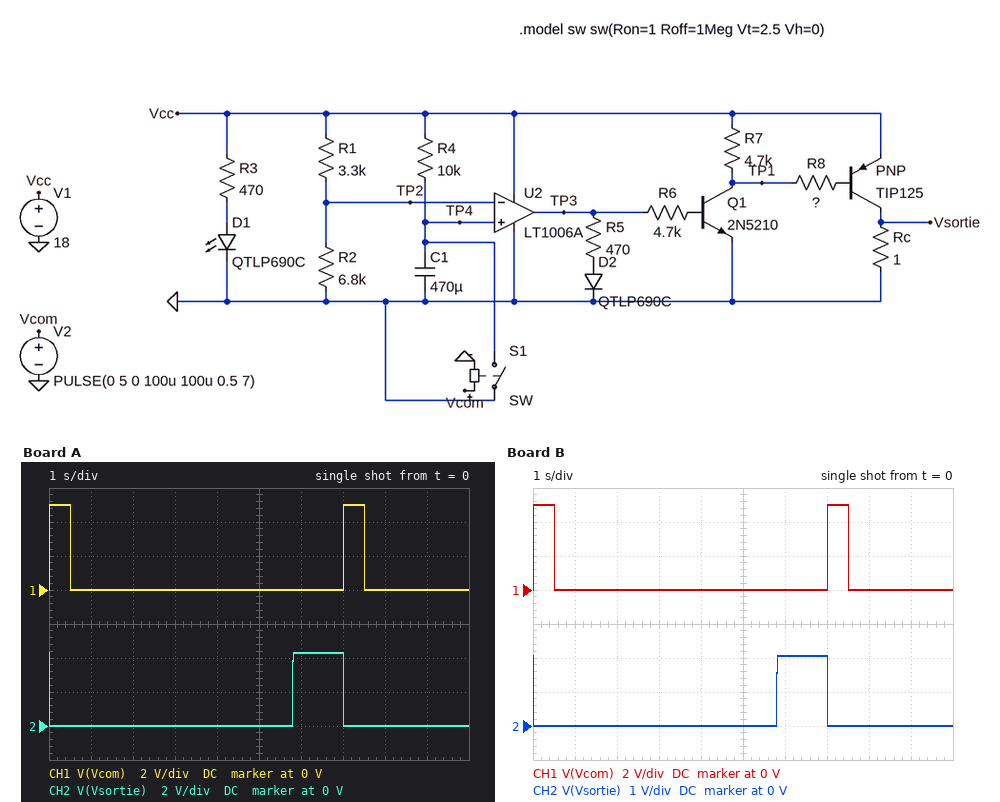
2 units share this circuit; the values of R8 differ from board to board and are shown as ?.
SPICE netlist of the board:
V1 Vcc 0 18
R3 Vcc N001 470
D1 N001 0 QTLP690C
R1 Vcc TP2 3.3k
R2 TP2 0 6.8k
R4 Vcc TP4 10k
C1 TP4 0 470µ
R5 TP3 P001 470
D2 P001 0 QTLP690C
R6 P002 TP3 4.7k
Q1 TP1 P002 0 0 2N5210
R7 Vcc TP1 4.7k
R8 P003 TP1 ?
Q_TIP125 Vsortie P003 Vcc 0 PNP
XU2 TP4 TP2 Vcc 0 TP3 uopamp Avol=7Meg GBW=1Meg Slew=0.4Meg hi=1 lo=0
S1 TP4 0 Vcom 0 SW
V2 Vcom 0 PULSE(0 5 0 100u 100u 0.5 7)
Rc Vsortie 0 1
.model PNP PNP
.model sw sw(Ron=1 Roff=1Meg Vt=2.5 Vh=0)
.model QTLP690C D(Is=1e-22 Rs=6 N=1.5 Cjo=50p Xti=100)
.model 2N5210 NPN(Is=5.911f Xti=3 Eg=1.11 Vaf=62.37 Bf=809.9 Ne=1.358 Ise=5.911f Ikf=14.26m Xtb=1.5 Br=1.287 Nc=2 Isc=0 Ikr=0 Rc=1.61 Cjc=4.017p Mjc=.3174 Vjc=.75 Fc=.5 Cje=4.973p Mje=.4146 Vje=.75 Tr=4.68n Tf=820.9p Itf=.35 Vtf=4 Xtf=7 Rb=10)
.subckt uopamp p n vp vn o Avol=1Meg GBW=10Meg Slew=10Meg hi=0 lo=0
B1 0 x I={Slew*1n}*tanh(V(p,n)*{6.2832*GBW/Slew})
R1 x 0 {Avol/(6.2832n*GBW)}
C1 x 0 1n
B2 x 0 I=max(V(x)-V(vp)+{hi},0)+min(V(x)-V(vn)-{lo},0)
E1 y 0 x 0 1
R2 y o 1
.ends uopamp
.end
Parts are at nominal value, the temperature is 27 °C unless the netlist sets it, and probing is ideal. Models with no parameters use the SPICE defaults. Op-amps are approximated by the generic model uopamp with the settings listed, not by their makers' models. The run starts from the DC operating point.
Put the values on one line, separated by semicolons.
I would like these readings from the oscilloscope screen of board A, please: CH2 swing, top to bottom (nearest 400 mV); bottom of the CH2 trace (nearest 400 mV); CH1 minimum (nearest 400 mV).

4.4 V; 0 V; 0 V
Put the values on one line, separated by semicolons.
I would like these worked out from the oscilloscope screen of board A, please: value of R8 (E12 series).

390 Ω
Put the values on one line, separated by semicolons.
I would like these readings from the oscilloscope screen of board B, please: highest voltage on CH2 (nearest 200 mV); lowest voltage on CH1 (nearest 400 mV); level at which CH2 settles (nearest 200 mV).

2.0 V; 0 V; 0 V
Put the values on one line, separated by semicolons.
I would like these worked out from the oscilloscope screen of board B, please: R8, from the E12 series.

820 Ω
